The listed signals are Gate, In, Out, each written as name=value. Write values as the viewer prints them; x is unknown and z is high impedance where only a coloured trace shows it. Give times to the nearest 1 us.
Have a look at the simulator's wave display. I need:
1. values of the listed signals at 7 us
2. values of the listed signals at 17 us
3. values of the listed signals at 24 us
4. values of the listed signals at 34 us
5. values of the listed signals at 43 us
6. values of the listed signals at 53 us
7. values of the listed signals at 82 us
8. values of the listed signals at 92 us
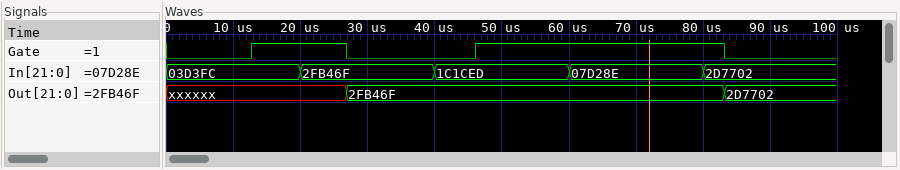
Gate=0, In=03D3FC, Out=xxxxxx
Gate=1, In=03D3FC, Out=xxxxxx
Gate=1, In=2FB46F, Out=xxxxxx
Gate=0, In=2FB46F, Out=2FB46F
Gate=0, In=1C1CED, Out=2FB46F
Gate=1, In=1C1CED, Out=2FB46F
Gate=1, In=2D7702, Out=2FB46F
Gate=0, In=2D7702, Out=2D7702
